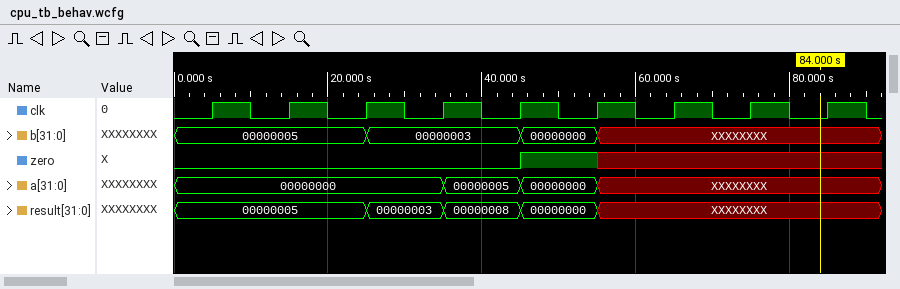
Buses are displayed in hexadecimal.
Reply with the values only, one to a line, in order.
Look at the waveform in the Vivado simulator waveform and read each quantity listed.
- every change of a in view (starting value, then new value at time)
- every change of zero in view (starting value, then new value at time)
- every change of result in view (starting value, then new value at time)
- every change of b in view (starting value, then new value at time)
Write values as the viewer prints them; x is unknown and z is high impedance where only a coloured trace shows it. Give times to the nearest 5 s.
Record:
00000000, 00000005 at 35 s, 00000000 at 45 s, XXXXXXXX at 55 s
0, 1 at 45 s, x at 55 s
00000005, 00000003 at 25 s, 00000008 at 35 s, 00000000 at 45 s, XXXXXXXX at 55 s
00000005, 00000003 at 25 s, 00000000 at 45 s, XXXXXXXX at 55 s
